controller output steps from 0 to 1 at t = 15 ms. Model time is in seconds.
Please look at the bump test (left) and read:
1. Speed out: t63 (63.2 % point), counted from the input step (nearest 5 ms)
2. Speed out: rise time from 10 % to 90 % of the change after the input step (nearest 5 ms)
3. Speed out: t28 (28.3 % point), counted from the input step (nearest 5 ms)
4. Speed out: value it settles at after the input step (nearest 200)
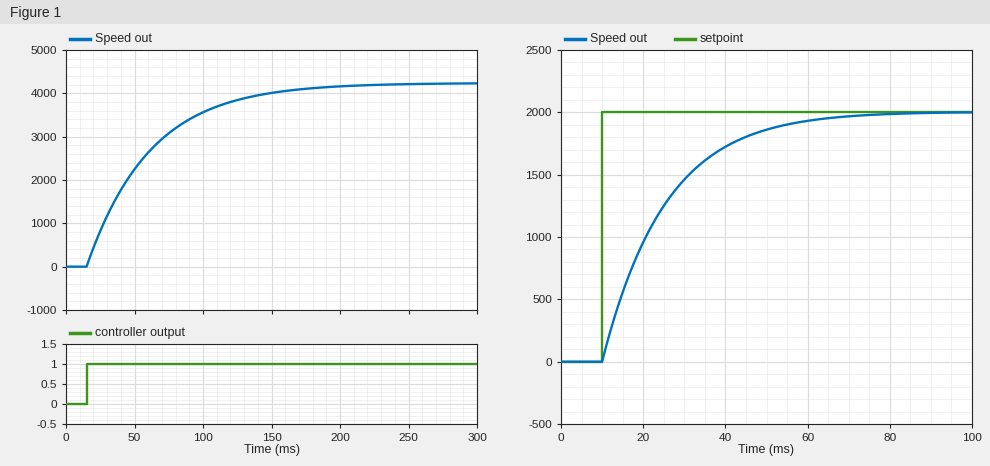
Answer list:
45 ms
100 ms
15 ms
4200
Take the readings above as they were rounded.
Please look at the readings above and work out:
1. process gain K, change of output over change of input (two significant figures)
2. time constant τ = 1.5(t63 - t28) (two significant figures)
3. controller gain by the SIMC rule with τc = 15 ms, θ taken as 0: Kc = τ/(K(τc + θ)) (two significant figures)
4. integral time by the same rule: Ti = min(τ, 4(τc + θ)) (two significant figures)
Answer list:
4200
45 ms
0.00071
45 ms
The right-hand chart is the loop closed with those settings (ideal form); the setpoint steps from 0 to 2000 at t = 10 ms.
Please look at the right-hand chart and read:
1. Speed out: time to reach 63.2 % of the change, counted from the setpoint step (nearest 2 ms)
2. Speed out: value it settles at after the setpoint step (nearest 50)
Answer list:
16 ms
2000
